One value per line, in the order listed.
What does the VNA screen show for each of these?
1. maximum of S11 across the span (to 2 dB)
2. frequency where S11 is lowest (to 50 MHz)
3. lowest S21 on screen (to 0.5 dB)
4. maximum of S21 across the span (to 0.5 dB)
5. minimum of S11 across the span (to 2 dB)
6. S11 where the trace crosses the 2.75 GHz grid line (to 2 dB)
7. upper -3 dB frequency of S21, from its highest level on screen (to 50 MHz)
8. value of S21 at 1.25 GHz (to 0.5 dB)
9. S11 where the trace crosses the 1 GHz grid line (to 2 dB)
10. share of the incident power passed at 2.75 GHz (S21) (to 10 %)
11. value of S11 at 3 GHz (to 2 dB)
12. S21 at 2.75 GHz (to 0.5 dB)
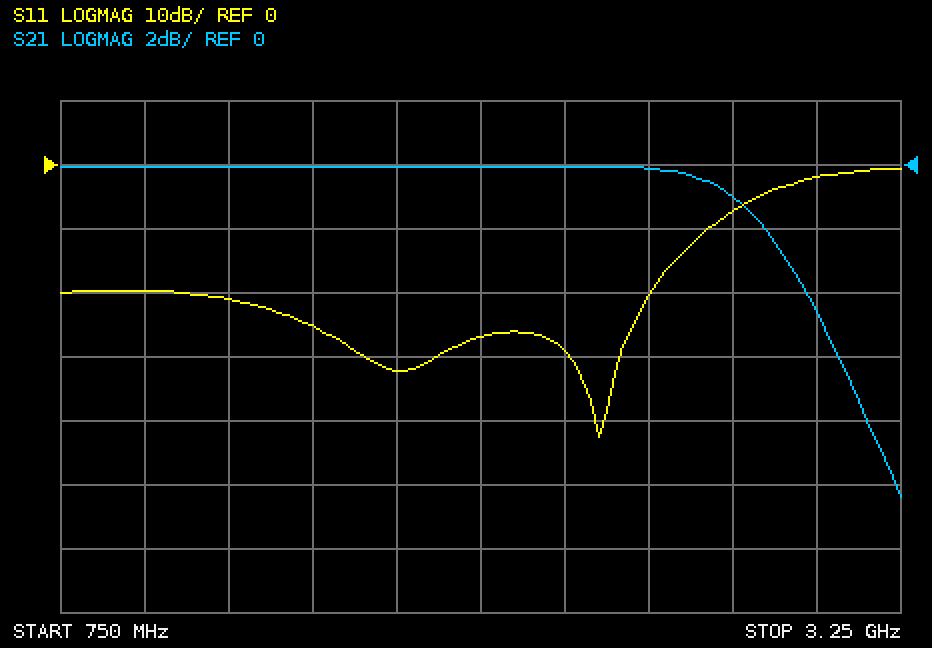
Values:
0 dB
2.35 GHz
-10.5 dB
0.0 dB
-42 dB
-8 dB
2.90 GHz
0.0 dB
-20 dB
80 %
-2 dB
-1.0 dB
